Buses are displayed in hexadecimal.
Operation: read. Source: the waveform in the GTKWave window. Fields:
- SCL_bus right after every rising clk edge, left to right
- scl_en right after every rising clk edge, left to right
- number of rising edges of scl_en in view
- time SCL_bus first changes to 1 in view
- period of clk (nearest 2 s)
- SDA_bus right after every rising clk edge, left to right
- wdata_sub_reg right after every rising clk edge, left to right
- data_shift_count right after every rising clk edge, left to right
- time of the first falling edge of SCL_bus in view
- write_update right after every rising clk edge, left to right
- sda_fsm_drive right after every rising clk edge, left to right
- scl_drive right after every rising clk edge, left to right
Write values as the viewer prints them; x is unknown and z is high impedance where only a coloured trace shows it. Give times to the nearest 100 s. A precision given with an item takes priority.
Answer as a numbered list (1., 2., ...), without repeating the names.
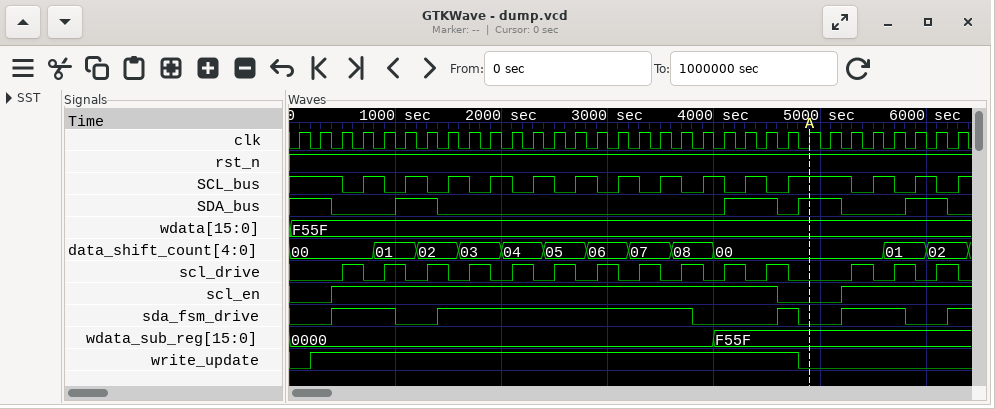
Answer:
1. 1 1 0 1 0 1 0 1 0 1 0 1 0 1 0 1 0 1 0 1 0 1 0 1 1 1 0 1 0 1 0 1
2. 0 0 1 1 1 1 1 1 1 1 1 1 1 1 1 1 1 1 1 1 1 1 1 0 0 0 1 1 1 1 1 1
3. 2
4. 700 s
5. 200 s
6. 1 1 0 0 0 1 1 0 0 0 0 0 0 0 0 0 0 0 0 0 1 1 1 0 1 1 0 0 0 1 1 0
7. 0000, 0000, 0000, 0000, 0000, 0000, 0000, 0000, 0000, 0000, 0000, 0000, 0000, 0000, 0000, 0000, 0000, 0000, 0000, 0000, F55F, F55F, F55F, F55F, F55F, F55F, F55F, F55F, F55F, F55F, F55F, F55F
8. 00, 00, 00, 00, 01, 01, 02, 02, 03, 03, 04, 04, 05, 05, 06, 06, 07, 07, 08, 08, 00, 00, 00, 00, 00, 00, 00, 00, 01, 01, 02, 02
9. 500 s
10. 0 1 1 1 1 1 1 1 1 1 1 1 1 1 1 1 1 1 1 1 1 1 1 1 0 0 0 0 0 0 0 0
11. 0 0 1 1 1 0 0 1 1 1 1 1 1 1 1 1 1 1 1 0 0 0 0 1 0 0 1 1 1 0 0 1
12. 0 0 1 0 1 0 1 0 1 0 1 0 1 0 1 0 1 0 1 0 1 0 1 0 0 0 1 0 1 0 1 0
